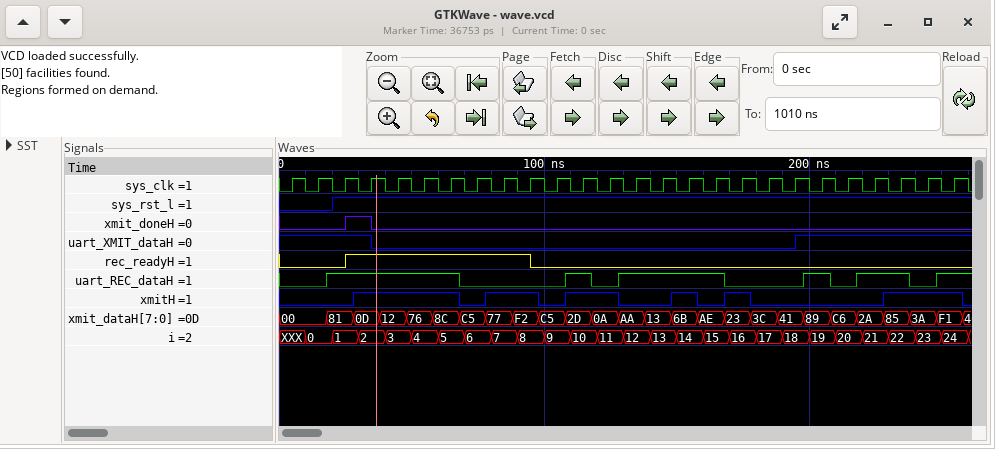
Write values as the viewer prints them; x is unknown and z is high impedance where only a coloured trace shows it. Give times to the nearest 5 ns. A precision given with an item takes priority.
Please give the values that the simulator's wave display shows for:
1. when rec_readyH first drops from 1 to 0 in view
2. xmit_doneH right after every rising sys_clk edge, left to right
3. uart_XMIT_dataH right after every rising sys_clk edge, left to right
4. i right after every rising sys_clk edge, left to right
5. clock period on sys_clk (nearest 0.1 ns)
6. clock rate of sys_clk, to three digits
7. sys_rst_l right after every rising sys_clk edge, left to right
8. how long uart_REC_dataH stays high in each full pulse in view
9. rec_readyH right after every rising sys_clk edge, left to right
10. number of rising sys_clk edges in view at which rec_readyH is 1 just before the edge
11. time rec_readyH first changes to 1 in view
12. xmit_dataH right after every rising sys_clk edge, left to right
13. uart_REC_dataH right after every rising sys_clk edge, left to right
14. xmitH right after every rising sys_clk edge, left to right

95 ns
0 0 1 0 0 0 0 0 0 0 0 0 0 0 0 0 0 0 0 0 0 0 0 0 0 0
1 1 1 0 0 0 0 0 0 0 0 0 0 0 0 0 0 0 0 1 1 1 1 1 1 1
XXX, 0, 1, 2, 3, 4, 5, 6, 7, 8, 9, 10, 11, 12, 13, 14, 15, 16, 17, 18, 19, 20, 21, 22, 23, 24
10 ns
100 MHz
0 0 1 1 1 1 1 1 1 1 1 1 1 1 1 1 1 1 1 1 1 1 1 1 1 1
50 ns, 10 ns, 40 ns, 10 ns, 20 ns
0 0 1 1 1 1 1 1 1 0 0 0 0 0 0 0 0 0 0 0 0 0 0 0 0 0
7
25 ns
00, 00, 81, 0D, 12, 76, 8C, C5, 77, F2, C5, 2D, 0A, AA, 13, 6B, AE, 23, 3C, 41, 89, C6, 2A, 85, 3A, F1
0 0 1 1 1 1 1 0 0 0 0 1 0 1 1 1 1 0 0 0 1 0 1 1 0 1
0 0 0 1 1 1 1 0 1 1 0 1 1 0 0 1 0 1 0 0 0 0 0 1 1 1
